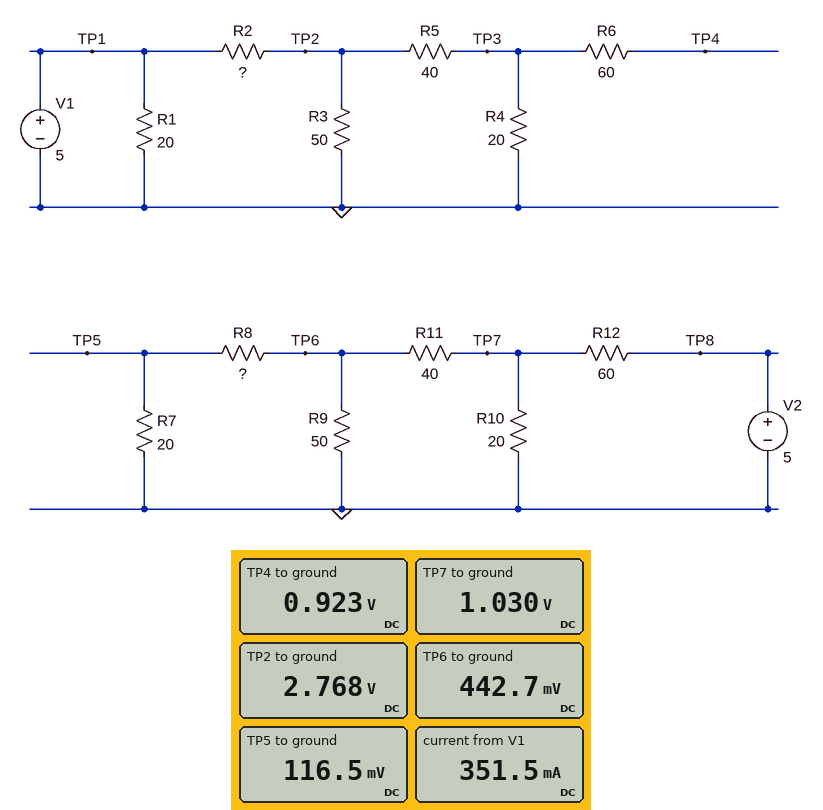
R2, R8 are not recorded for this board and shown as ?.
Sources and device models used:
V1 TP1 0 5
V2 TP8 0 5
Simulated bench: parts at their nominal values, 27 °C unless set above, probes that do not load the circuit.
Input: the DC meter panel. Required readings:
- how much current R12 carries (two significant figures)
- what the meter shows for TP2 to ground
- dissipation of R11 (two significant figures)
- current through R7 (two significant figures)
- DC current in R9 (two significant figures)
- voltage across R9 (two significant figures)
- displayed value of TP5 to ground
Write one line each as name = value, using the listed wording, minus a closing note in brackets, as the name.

how much current R12 carries = 66 mA
what the meter shows for TP2 to ground = 2.768 V
dissipation of R11 = 8.6 mW
current through R7 = 5.8 mA
DC current in R9 = 8.9 mA
voltage across R9 = 440 mV
displayed value of TP5 to ground = 116.5 mV
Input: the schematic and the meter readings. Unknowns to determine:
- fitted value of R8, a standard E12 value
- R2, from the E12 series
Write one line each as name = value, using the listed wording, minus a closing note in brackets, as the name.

fitted value of R8, a standard E12 value = 56 Ω
R2, from the E12 series = 22 Ω
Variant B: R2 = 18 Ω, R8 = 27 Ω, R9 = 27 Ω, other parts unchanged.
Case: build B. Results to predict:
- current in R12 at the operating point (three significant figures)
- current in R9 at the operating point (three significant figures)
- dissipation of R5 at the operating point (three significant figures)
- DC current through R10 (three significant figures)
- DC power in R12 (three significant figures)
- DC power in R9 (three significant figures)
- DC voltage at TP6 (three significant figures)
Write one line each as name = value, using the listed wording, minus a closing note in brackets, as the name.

current in R12 at the operating point = 66.8 mA
current in R9 at the operating point = 11.0 mA
dissipation of R5 at the operating point = 101 mW
DC current through R10 = 49.5 mA
DC power in R12 = 268 mW
DC power in R9 = 3.27 mW
DC voltage at TP6 = 297 mV
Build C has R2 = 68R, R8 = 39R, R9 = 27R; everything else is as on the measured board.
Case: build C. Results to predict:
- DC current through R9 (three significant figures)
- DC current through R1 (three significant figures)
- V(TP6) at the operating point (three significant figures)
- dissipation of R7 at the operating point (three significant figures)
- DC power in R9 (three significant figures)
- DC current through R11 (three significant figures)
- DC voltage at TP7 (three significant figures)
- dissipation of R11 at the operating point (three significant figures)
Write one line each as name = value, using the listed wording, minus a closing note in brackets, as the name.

DC current through R9 = 11.7 mA
DC current through R1 = 250 mA
V(TP6) at the operating point = 315 mV
dissipation of R7 at the operating point = 570 µW
DC power in R9 = 3.67 mW
DC current through R11 = 17.0 mA
DC voltage at TP7 = 995 mV
dissipation of R11 at the operating point = 11.6 mW
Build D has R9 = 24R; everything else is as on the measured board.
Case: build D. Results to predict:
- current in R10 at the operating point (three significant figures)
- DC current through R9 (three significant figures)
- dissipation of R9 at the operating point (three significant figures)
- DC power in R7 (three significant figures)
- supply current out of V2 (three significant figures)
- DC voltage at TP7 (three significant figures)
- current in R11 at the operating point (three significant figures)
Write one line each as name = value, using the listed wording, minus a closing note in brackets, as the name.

current in R10 at the operating point = 49.7 mA
DC current through R9 = 13.0 mA
dissipation of R9 at the operating point = 4.04 mW
DC power in R7 = 336 µW
supply current out of V2 = 66.8 mA
DC voltage at TP7 = 994 mV
current in R11 at the operating point = 17.1 mA
